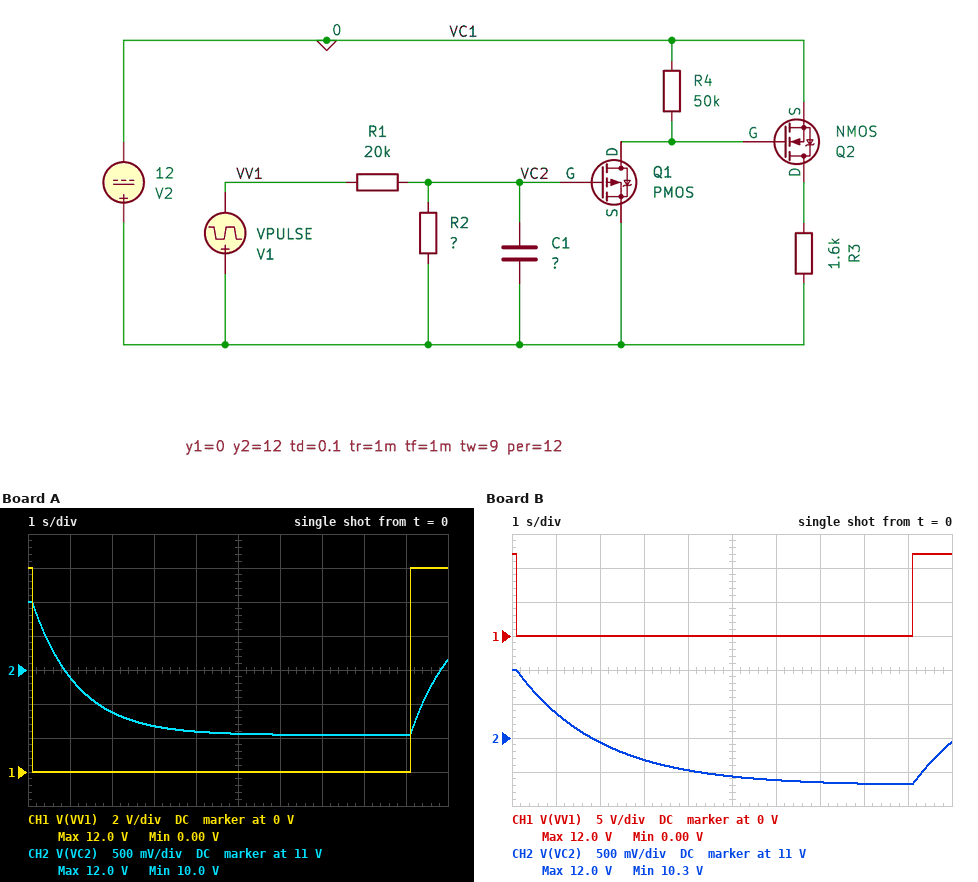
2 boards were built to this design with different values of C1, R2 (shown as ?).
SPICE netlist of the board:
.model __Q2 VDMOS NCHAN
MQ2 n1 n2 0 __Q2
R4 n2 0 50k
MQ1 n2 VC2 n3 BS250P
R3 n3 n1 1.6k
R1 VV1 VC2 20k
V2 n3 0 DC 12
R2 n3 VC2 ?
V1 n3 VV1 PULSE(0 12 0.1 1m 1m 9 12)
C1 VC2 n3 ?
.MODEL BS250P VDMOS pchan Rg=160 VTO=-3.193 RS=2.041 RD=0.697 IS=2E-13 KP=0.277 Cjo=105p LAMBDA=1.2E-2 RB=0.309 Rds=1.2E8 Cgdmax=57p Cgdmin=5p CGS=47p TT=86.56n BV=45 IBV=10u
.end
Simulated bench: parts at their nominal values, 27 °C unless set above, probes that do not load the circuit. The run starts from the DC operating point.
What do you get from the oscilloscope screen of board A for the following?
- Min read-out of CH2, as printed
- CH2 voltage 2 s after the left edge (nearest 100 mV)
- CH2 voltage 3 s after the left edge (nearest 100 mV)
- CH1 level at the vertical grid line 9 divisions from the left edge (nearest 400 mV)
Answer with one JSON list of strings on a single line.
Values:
["10.0 V", "10.4 V", "10.2 V", "0 V"]
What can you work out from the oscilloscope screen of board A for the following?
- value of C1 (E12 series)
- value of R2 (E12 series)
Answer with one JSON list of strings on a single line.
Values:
["330 µF", "3.9 kΩ"]
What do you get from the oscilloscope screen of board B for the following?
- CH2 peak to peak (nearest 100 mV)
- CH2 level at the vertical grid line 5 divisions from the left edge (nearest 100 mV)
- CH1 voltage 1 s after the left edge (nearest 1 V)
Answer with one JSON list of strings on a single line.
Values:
["1.7 V", "10.4 V", "0 V"]
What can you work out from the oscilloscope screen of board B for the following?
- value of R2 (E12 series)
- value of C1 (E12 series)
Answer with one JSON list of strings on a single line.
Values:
["3.3 kΩ", "680 µF"]
